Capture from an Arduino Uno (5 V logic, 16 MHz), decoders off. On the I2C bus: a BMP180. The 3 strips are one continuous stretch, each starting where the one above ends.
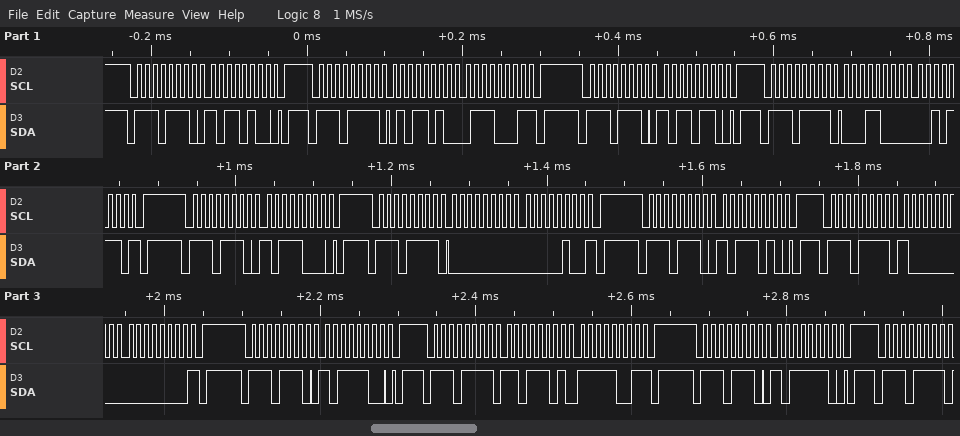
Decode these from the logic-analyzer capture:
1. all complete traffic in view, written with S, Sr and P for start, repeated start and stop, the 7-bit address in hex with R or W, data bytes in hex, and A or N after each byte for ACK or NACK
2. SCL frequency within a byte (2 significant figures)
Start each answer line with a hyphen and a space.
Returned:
- S 77W A B4 A P S 77R A 5A A 71 N P S 77W A B6 A P S 77R A 18 A 2E N P S 77W A B8 A P S 77R A 00 A 04 N P S 77W A BA A P S 77R A 80 A 00 N P S 77W A BC A P S 77R A DD A F9 N P S 77W A BE A P S 77R A
- 100 kHz
